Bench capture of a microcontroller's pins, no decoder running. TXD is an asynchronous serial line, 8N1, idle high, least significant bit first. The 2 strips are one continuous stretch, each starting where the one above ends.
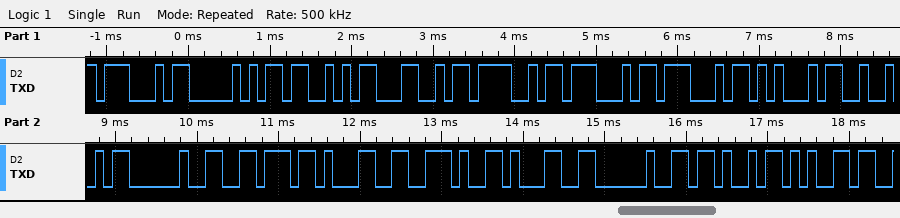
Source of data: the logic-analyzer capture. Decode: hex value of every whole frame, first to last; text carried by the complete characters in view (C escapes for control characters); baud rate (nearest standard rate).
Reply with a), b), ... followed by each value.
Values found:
a) 47 50 53 4C 4F 47 47 45 52 20 76 31 2E 31 20 4B 65
b) "GPSLOGGER v1.1 Ke"
c) 9600 baud
